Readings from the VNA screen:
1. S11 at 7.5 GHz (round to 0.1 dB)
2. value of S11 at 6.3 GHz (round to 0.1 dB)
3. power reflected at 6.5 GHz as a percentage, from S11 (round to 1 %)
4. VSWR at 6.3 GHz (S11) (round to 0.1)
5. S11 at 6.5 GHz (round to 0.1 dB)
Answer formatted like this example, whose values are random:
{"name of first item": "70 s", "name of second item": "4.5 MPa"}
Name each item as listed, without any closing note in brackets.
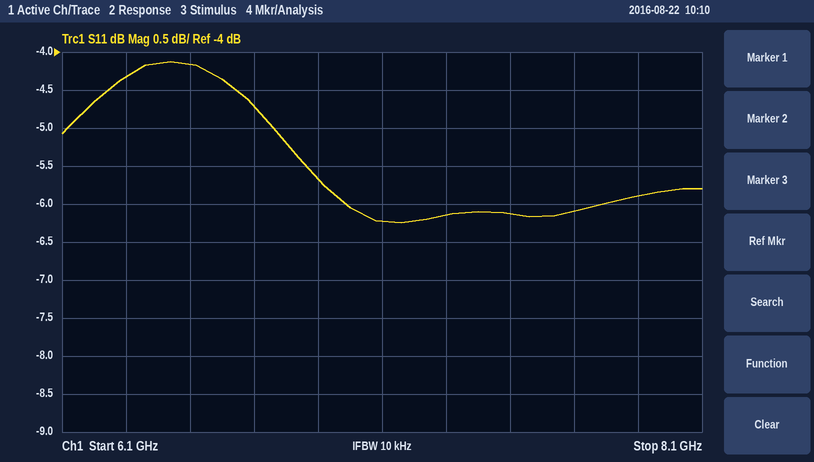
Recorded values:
{"S11 at 7.5 GHz": "-6.1 dB", "value of S11 at 6.3 GHz": "-4.3 dB", "power reflected at 6.5 GHz as a percentage, from S11": "38 %", "VSWR at 6.3 GHz (S11)": "4.1", "S11 at 6.5 GHz": "-4.2 dB"}
